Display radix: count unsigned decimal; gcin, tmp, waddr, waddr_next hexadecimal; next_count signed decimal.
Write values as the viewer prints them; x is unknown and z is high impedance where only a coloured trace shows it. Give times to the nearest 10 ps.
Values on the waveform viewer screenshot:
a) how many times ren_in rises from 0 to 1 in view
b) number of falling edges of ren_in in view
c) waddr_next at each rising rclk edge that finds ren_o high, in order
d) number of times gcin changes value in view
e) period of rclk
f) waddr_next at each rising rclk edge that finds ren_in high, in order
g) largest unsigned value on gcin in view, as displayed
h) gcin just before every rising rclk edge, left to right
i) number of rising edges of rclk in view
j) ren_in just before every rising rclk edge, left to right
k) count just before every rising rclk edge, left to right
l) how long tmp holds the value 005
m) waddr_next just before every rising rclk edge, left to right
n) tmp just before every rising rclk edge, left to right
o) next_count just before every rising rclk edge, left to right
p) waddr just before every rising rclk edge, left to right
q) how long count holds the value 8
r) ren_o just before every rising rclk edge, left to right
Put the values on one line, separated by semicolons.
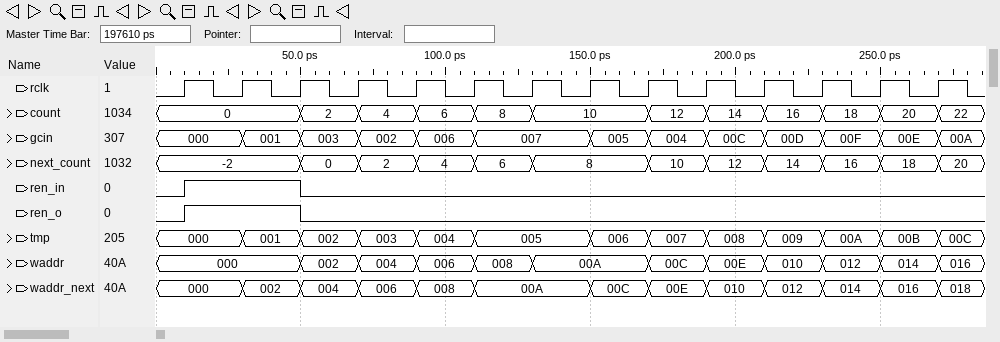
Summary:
1; 1; 000, 002; 12; 20 ps; 000, 002; 00F; 000, 000, 001, 003, 002, 006, 007, 007, 005, 004, 00C, 00D, 00F, 00E; 14; 0 1 1 0 0 0 0 0 0 0 0 0 0 0; 0, 0, 0, 2, 4, 6, 8, 10, 10, 12, 14, 16, 18, 20; 40 ps; 000, 000, 002, 004, 006, 008, 00A, 00A, 00C, 00E, 010, 012, 014, 016; 000, 000, 001, 002, 003, 004, 005, 005, 006, 007, 008, 009, 00A, 00B; -2, -2, -2, 0, 2, 4, 6, 8, 8, 10, 12, 14, 16, 18; 000, 000, 000, 002, 004, 006, 008, 00A, 00A, 00C, 00E, 010, 012, 014; 20 ps; 0 1 1 0 0 0 0 0 0 0 0 0 0 0
